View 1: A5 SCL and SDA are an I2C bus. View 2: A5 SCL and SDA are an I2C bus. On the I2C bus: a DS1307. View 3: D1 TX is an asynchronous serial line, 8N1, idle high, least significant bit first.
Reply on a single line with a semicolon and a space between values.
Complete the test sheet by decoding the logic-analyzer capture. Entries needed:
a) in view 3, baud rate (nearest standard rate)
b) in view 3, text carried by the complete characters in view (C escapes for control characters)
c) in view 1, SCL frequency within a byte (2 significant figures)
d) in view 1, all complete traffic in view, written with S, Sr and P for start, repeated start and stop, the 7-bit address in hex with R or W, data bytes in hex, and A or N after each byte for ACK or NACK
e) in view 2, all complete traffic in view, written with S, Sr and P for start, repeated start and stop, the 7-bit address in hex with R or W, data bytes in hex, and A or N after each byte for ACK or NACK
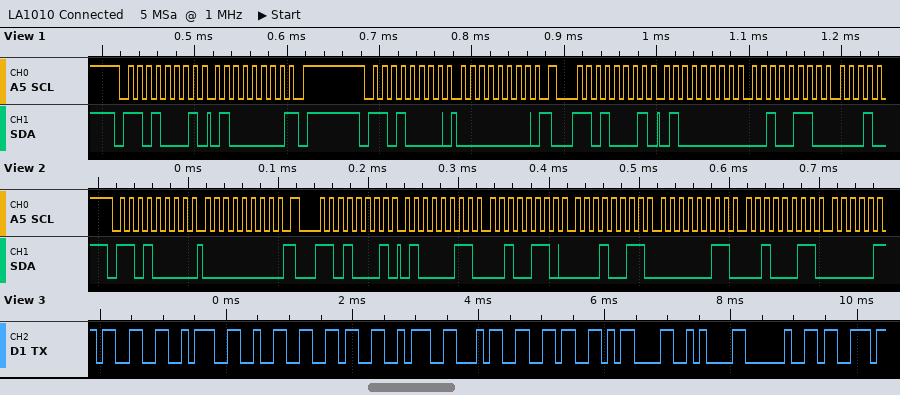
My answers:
9600 baud; "3:26:46\r\n s"; 100 kHz; S 68R A 40 N P S 68W A 00 A Sr 68R A 40 A 26 A; S 68W A 00 A Sr 68R A 43 A 26 A 13 A 03 A 23 A
